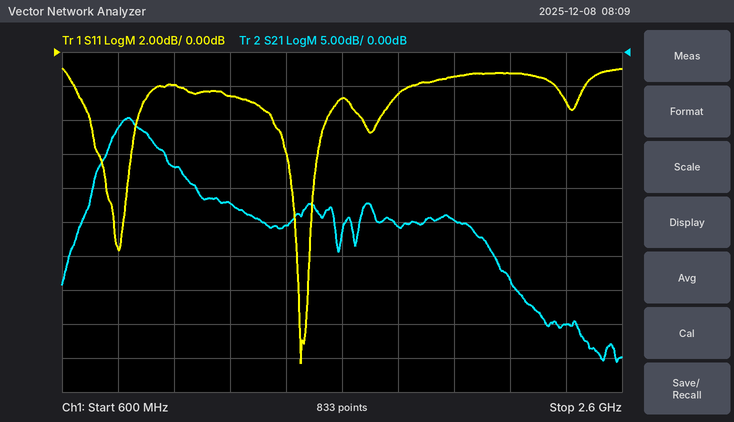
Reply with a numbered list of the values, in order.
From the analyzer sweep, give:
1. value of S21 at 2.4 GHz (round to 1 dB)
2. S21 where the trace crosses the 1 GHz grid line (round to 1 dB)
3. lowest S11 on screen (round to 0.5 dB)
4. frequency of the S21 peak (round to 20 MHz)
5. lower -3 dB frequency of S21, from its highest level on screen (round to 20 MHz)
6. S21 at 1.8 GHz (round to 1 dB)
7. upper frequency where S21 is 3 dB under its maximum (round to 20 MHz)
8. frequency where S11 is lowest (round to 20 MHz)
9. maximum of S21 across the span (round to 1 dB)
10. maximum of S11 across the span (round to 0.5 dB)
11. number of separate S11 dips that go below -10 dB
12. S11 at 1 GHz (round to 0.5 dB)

1. -40 dB
2. -17 dB
3. -18.5 dB
4. 840 MHz
5. 780 MHz
6. -26 dB
7. 920 MHz
8. 1.46 GHz
9. -10 dB
10. -1.0 dB
11. 2
12. -2.0 dB
